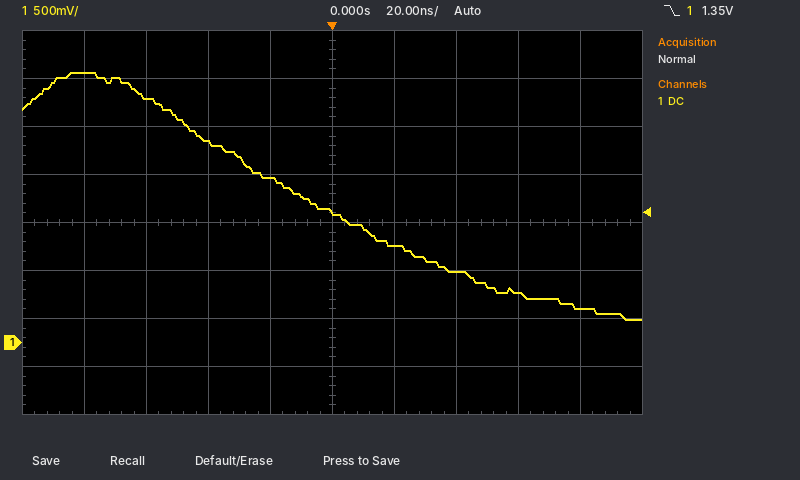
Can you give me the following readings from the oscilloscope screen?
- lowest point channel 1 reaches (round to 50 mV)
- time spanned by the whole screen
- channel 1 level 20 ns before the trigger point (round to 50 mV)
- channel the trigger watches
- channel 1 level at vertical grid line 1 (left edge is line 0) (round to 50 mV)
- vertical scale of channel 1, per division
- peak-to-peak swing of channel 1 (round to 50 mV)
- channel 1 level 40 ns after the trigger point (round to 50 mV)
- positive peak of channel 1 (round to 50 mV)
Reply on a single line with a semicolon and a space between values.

250 mV; 200 ns; 1.70 V; channel 1; 2.80 V; 500 mV; 2.55 V; 750 mV; 2.80 V
